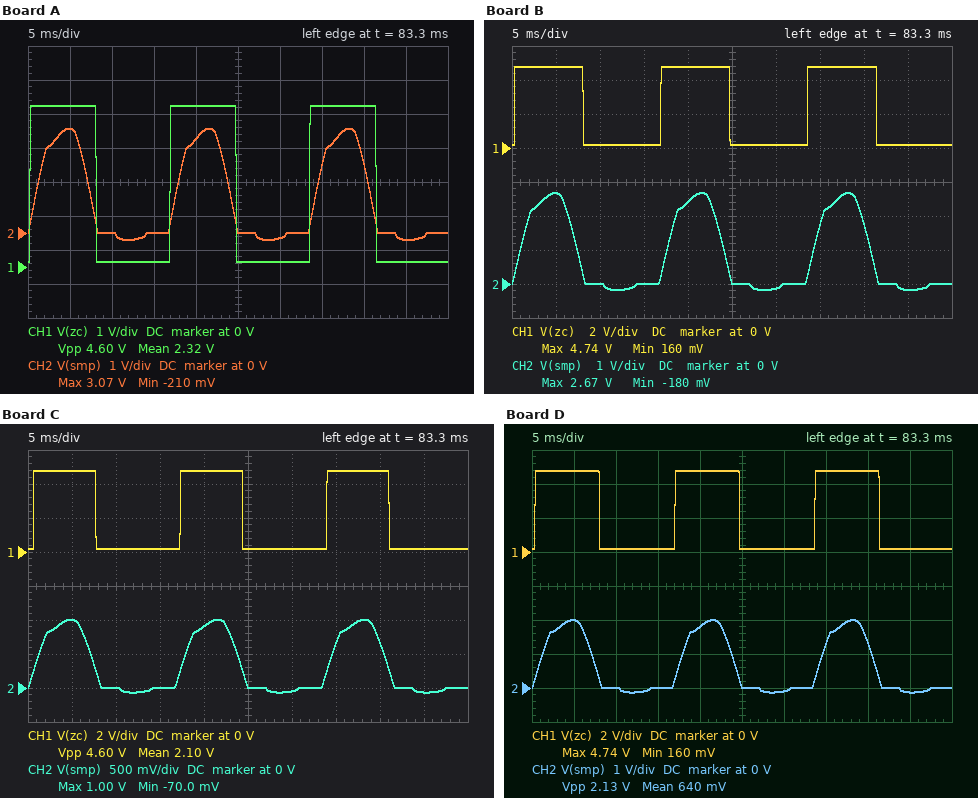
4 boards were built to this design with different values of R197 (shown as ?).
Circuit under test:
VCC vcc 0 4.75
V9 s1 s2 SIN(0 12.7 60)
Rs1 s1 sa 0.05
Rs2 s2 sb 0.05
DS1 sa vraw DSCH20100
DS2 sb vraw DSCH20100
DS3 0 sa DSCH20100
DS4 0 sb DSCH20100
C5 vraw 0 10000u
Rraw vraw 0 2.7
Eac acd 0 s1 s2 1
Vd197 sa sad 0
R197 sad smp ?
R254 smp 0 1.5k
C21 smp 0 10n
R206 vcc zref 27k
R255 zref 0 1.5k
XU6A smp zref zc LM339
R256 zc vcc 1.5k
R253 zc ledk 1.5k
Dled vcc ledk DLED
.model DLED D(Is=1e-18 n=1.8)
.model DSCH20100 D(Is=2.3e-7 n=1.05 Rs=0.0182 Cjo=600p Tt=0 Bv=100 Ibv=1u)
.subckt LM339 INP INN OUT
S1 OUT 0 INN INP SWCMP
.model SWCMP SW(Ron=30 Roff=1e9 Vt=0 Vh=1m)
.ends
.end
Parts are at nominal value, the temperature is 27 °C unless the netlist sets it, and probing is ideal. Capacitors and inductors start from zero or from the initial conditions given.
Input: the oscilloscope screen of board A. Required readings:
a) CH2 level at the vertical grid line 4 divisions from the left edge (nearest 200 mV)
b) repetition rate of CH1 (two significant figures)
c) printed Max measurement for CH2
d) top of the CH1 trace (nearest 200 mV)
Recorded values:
2.8 V
60 Hz
3.07 V
4.8 V
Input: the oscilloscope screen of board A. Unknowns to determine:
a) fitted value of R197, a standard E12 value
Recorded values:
3.9 kΩ
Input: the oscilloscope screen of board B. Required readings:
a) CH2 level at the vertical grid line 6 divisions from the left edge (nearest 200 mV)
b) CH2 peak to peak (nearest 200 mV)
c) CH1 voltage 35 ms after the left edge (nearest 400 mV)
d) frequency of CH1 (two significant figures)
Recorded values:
-200 mV
2.8 V
4.8 V
60 Hz
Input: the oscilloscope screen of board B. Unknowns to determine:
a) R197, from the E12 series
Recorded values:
4.7 kΩ
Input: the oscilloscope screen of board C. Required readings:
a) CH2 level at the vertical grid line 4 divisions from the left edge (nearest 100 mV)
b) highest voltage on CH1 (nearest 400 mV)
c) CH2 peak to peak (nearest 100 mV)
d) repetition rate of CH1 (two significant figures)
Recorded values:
900 mV
4.8 V
1.1 V
60 Hz
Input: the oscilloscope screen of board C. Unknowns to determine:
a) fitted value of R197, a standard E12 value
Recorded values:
15 kΩ
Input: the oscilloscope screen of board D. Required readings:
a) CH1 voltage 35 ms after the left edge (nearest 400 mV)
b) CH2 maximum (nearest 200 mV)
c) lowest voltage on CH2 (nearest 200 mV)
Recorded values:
4.8 V
2.0 V
-200 mV
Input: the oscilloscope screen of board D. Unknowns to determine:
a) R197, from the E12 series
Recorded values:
6.8 kΩ
